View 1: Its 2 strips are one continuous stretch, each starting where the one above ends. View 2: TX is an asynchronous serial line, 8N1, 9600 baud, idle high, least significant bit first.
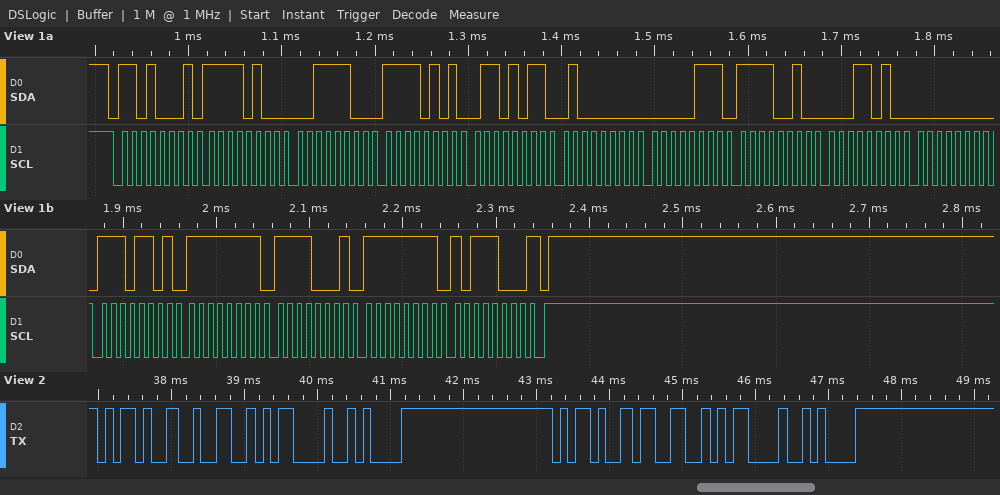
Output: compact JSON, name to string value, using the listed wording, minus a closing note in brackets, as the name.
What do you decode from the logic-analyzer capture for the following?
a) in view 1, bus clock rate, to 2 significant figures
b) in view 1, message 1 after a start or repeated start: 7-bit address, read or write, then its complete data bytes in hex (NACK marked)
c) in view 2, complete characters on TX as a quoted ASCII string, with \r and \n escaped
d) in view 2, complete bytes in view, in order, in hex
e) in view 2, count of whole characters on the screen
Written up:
{"in view 1, bus clock rate, to 2 significant figures": "100 kHz", "in view 1, message 1 after a start or repeated start: 7-bit address, read or write, then its complete data bytes in hex": "0x68 read: F4 3C F5 6B 40 07 F2 1A 00 ED FF F1 FF B8 NACK", "in view 2, complete characters on TX as a quoted ASCII string, with \\r and \\n escaped": "\"-2\\r\\n-3\\r\\n\"", "in view 2, complete bytes in view, in order, in hex": "2D 32 0D 0A 2D 33 0D 0A", "in view 2, count of whole characters on the screen": "8"}
